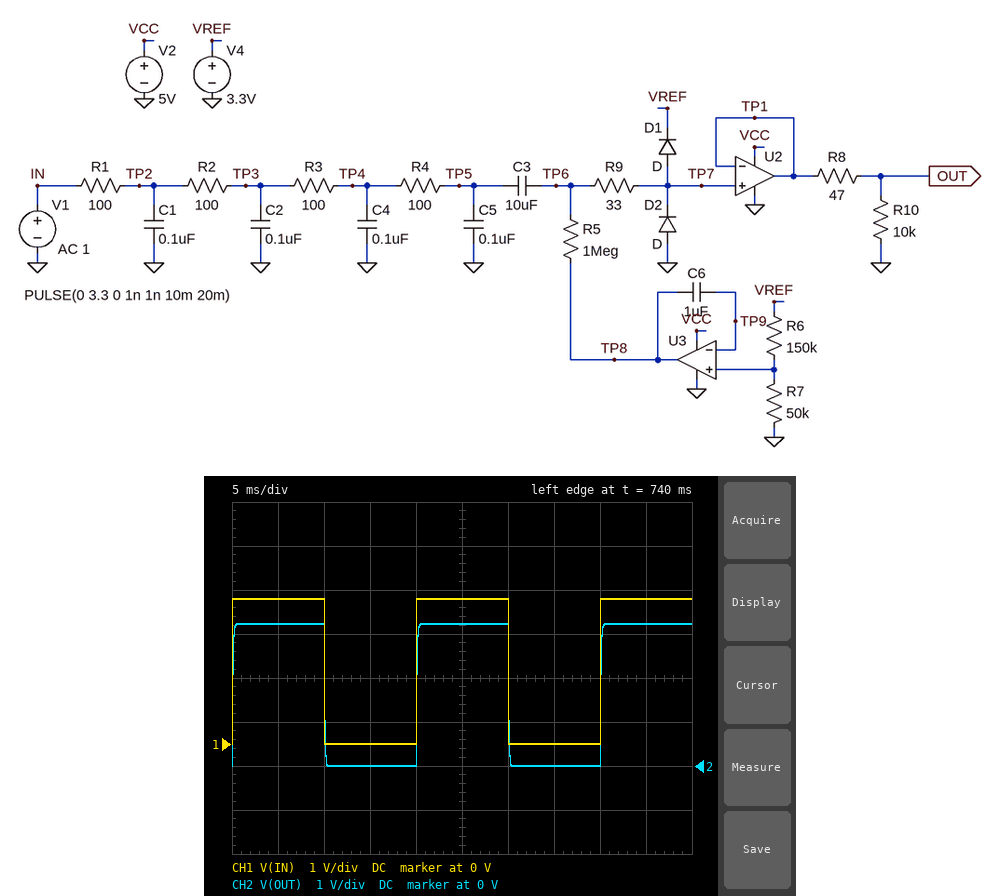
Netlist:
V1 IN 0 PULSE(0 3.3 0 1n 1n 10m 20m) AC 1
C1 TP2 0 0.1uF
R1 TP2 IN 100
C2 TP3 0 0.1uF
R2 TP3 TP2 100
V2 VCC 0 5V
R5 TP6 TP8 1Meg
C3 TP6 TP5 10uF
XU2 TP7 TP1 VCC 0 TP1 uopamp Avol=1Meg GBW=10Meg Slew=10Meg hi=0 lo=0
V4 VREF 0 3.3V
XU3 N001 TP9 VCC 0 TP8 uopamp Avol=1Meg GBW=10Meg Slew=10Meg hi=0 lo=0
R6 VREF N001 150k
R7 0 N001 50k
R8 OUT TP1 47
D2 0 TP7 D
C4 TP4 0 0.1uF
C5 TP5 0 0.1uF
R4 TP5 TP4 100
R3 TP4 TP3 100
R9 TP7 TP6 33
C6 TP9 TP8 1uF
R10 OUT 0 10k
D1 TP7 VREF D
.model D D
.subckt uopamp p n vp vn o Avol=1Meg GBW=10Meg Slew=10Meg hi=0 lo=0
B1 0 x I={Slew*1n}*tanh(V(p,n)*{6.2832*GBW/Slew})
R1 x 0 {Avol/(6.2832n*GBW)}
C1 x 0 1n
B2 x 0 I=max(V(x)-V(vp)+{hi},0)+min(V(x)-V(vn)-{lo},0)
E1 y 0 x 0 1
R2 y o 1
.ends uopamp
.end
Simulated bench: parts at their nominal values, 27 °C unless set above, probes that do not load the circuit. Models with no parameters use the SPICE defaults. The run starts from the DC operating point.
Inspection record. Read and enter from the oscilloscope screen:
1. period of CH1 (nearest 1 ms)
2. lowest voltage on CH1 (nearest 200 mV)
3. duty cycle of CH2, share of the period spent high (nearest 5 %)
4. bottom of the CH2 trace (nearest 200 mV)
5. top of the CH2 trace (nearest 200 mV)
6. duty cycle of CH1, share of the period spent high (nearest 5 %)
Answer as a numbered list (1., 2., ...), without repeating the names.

1. 20 ms
2. 0 V
3. 50 %
4. 0 V
5. 3.2 V
6. 50 %
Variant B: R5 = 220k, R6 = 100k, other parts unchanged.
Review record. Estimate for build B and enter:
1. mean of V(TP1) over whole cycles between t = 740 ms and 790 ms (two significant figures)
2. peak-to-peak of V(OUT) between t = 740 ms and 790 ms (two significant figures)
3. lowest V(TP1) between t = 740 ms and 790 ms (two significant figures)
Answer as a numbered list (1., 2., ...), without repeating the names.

1. 1.6 V
2. 3.1 V
3. -7.6 mV
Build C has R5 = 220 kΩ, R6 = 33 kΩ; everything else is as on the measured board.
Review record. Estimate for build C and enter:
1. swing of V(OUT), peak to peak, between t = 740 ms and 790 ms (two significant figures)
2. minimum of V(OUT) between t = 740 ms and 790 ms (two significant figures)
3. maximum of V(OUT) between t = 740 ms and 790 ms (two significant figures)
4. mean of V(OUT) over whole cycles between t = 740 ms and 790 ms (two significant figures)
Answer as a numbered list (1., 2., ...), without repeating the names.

1. 3.3 V
2. 95 mV
3. 3.4 V
4. 1.7 V
